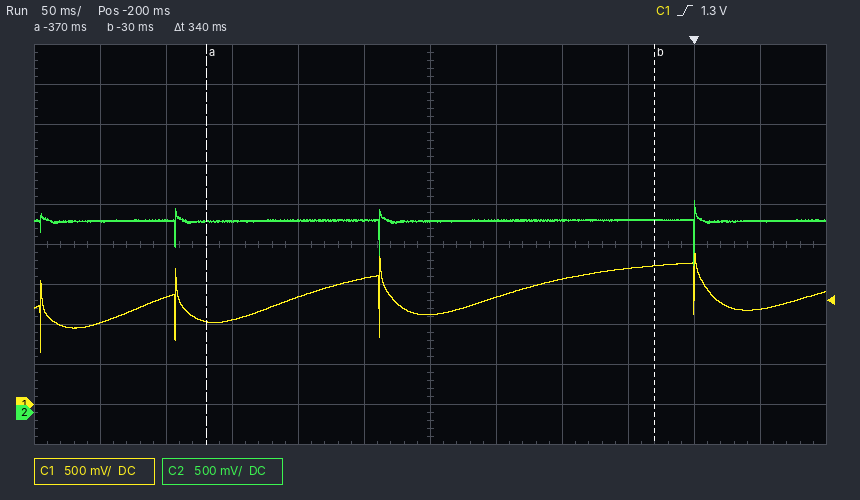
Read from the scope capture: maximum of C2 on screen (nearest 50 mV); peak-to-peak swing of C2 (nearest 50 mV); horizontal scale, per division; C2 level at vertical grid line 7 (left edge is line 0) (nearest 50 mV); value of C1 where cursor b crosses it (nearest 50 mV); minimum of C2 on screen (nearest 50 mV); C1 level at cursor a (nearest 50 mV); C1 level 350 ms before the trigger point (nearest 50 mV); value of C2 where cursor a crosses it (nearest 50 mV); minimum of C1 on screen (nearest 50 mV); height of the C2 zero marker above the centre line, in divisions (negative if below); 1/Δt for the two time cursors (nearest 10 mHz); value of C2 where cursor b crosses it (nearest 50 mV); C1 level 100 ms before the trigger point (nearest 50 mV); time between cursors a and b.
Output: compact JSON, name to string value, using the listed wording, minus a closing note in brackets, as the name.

{"maximum of C2 on screen": "2.65 V", "peak-to-peak swing of C2": "800 mV", "horizontal scale, per division": "50 ms", "C2 level at vertical grid line 7 (left edge is line 0)": "2.40 V", "value of C1 where cursor b crosses it": "1.75 V", "minimum of C2 on screen": "1.85 V", "C1 level at cursor a": "1.05 V", "C1 level 350 ms before the trigger point": "1.05 V", "value of C2 where cursor a crosses it": "2.40 V", "minimum of C1 on screen": "650 mV", "height of the C2 zero marker above the centre line, in divisions": "-4.2 div", "1/Δt for the two time cursors": "2.94 Hz", "value of C2 where cursor b crosses it": "2.40 V", "C1 level 100 ms before the trigger point": "1.55 V", "time between cursors a and b": "340 ms"}
